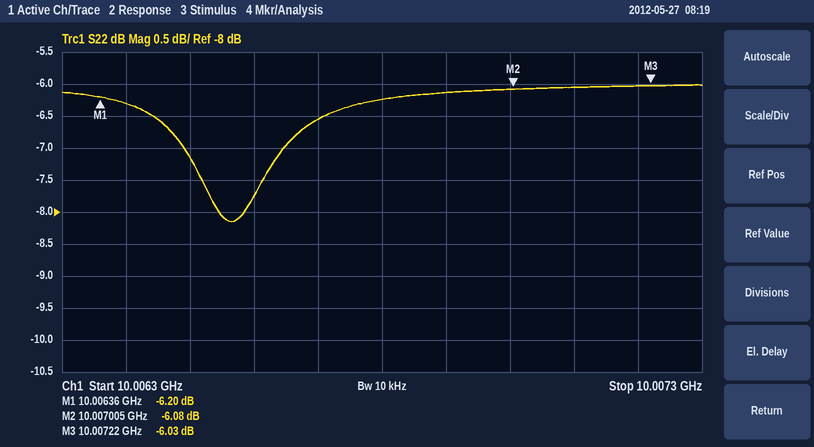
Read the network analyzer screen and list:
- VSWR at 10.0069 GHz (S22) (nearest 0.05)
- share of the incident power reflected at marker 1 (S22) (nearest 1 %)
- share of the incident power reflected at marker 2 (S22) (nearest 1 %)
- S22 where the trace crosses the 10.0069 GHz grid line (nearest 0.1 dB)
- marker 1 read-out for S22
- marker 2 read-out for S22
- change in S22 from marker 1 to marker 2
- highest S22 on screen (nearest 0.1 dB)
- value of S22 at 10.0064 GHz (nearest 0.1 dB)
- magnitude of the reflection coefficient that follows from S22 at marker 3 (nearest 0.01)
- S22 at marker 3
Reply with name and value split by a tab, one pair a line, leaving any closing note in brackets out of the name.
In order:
VSWR at 10.0069 GHz (S22)	2.95
share of the incident power reflected at marker 1 (S22)	24 %
share of the incident power reflected at marker 2 (S22)	25 %
S22 where the trace crosses the 10.0069 GHz grid line	-6.1 dB
marker 1 read-out for S22	-6.20 dB
marker 2 read-out for S22	-6.08 dB
change in S22 from marker 1 to marker 2	0.12 dB
highest S22 on screen	-6.0 dB
value of S22 at 10.0064 GHz	-6.3 dB
magnitude of the reflection coefficient that follows from S22 at marker 3	0.50
S22 at marker 3	-6.03 dB
